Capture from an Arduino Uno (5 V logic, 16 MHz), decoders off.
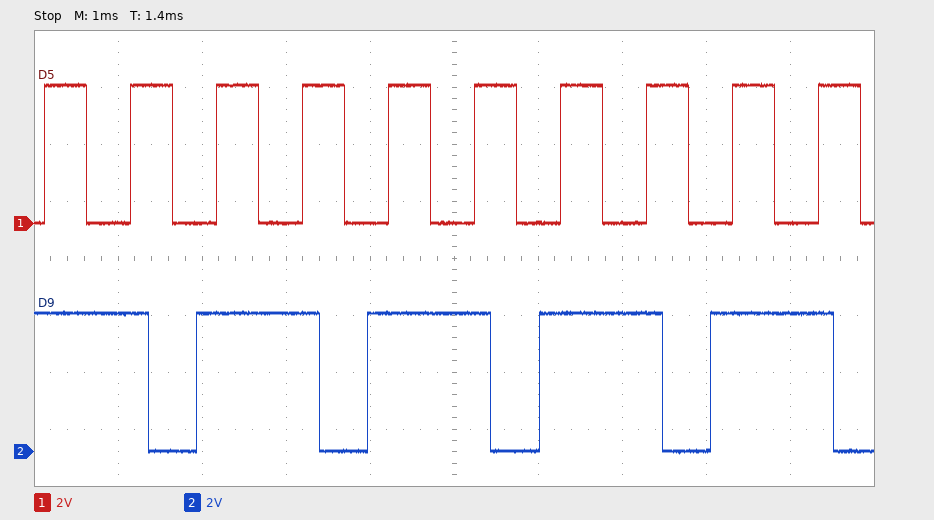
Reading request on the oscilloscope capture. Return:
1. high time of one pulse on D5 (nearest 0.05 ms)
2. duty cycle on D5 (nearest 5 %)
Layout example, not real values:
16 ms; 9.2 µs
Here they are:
0.50 ms; 50 %
